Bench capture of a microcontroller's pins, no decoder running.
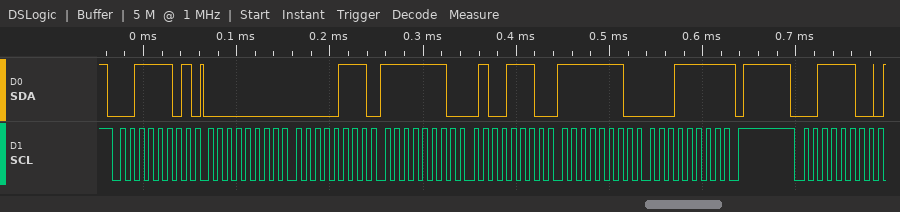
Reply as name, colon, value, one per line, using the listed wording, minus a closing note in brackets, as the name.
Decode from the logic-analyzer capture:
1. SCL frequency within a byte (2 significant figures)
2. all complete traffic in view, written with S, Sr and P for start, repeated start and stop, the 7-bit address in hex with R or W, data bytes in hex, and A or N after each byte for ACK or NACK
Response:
SCL frequency within a byte: 100 kHz
all complete traffic in view, written with S, Sr and P for start, repeated start and stop, the 7-bit address in hex with R or W, data bytes in hex, and A or N after each byte for ACK or NACK: S 1ER A 00 A 07 A FE A 4E A FE A 1F N P S 1EW A
